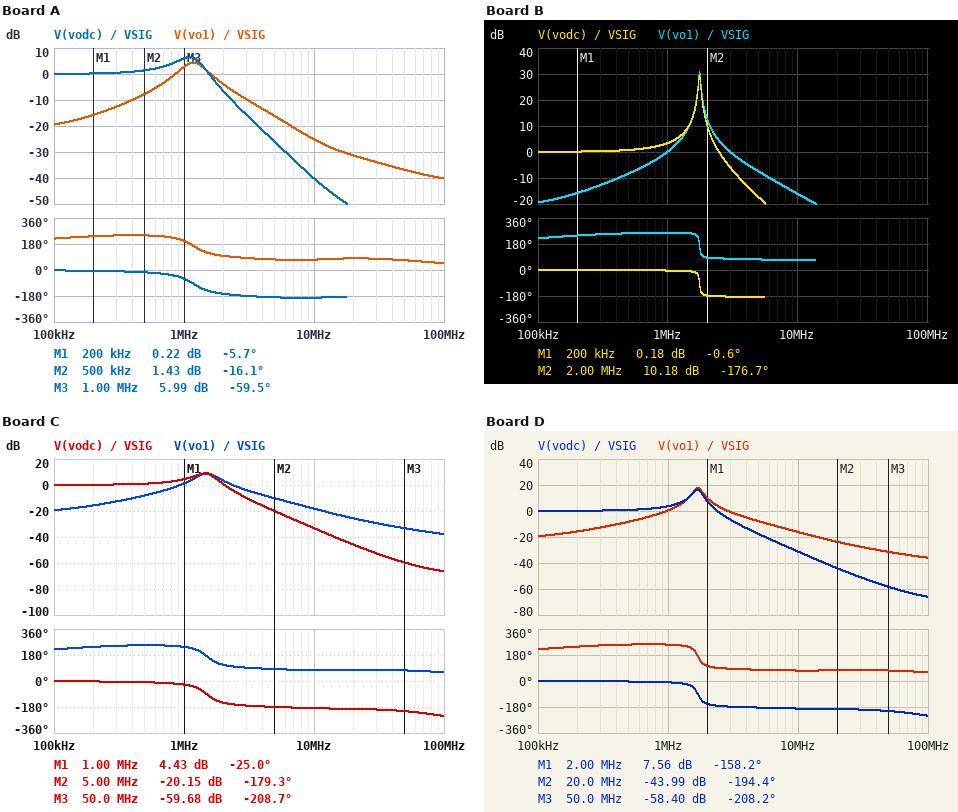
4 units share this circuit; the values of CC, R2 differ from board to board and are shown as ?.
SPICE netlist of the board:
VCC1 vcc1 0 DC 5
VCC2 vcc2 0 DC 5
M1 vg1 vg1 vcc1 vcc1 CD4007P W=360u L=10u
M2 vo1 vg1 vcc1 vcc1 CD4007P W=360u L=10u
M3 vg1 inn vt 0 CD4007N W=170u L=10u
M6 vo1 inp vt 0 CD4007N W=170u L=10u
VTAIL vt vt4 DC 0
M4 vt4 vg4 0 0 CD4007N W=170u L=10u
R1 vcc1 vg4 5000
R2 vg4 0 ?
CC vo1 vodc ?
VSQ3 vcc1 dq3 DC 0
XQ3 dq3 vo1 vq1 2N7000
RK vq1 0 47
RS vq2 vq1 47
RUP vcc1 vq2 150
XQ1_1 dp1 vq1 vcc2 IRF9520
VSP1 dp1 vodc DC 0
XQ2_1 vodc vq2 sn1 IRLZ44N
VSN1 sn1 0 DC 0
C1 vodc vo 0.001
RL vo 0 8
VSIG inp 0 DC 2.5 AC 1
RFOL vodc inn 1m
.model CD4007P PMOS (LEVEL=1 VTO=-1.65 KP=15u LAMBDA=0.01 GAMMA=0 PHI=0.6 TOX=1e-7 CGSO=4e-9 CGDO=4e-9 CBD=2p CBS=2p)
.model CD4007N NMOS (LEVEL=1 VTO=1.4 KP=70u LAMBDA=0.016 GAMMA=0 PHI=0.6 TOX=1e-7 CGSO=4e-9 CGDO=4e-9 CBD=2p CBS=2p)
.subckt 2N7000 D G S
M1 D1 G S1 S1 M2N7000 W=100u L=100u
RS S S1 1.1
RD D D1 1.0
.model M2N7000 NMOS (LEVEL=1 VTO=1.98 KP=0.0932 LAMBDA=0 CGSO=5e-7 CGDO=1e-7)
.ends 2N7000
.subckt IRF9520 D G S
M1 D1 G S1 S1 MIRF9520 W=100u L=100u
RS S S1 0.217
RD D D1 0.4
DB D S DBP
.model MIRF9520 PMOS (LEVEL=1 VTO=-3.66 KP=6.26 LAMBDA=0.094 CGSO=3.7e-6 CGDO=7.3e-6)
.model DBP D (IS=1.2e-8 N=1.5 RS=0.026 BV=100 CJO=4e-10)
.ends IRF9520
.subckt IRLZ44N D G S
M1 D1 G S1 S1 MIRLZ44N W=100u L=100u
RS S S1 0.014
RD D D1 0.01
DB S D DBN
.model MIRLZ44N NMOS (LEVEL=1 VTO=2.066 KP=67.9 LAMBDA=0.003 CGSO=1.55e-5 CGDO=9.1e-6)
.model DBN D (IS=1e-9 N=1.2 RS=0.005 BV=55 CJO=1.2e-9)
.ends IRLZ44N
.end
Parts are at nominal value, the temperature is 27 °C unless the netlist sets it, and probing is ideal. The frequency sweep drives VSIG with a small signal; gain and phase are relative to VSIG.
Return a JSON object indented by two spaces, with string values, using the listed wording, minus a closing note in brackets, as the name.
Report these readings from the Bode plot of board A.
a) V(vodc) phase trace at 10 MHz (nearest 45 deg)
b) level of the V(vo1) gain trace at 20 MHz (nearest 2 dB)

{
  "V(vodc) phase trace at 10 MHz": "-180 deg",
  "level of the V(vo1) gain trace at 20 MHz": "-32 dB"
}
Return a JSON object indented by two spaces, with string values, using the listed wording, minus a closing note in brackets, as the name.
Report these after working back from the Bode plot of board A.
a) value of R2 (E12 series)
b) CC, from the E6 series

{
  "value of R2": "3.3 kΩ",
  "CC, from the E6 series": "33 pF"
}
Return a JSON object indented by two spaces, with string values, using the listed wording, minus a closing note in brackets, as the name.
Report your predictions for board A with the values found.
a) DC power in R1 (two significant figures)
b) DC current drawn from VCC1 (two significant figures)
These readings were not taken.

{
  "DC power in R1": "1.8 mW",
  "DC current drawn from VCC1": "26 mA"
}
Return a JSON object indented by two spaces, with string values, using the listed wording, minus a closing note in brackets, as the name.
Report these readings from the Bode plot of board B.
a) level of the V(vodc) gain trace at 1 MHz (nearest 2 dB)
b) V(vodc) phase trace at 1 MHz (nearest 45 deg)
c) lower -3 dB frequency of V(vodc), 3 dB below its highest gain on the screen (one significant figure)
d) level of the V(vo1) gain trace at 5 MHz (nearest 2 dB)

{
  "level of the V(vodc) gain trace at 1 MHz": "4 dB",
  "V(vodc) phase trace at 1 MHz": "0 deg",
  "lower -3 dB frequency of V(vodc), 3 dB below its highest gain on the screen": "2 MHz",
  "level of the V(vo1) gain trace at 5 MHz": "-8 dB"
}
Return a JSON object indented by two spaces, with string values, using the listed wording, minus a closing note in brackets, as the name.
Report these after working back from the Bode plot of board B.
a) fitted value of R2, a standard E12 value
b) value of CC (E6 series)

{
  "fitted value of R2, a standard E12 value": "4.7 kΩ",
  "value of CC": "6.8 pF"
}
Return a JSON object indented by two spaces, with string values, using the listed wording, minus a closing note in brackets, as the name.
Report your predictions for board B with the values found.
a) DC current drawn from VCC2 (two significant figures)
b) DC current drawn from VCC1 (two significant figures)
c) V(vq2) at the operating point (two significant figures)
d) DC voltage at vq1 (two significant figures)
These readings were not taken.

{
  "DC current drawn from VCC2": "60 mA",
  "DC current drawn from VCC1": "27 mA",
  "V(vq2) at the operating point": "2.1 V",
  "DC voltage at vq1": "1.2 V"
}
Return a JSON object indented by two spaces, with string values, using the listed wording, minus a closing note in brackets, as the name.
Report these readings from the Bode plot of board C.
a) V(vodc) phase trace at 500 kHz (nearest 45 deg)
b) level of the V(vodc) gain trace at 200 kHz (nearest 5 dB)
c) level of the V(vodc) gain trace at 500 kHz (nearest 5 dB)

{
  "V(vodc) phase trace at 500 kHz": "0 deg",
  "level of the V(vodc) gain trace at 200 kHz": "0 dB",
  "level of the V(vodc) gain trace at 500 kHz": "0 dB"
}
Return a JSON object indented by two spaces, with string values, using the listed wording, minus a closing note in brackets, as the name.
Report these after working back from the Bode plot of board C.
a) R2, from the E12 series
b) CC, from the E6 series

{
  "R2, from the E12 series": "5.6 kΩ",
  "CC, from the E6 series": "33 pF"
}
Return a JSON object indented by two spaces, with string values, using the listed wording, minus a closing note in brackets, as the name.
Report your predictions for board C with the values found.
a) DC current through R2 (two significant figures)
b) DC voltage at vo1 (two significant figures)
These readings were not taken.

{
  "DC current through R2": "470 µA",
  "DC voltage at vo1": "3.6 V"
}
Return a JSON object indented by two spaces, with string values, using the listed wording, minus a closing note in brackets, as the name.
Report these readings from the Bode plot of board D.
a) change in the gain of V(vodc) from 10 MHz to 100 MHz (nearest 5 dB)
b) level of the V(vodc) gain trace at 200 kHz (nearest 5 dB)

{
  "change in the gain of V(vodc) from 10 MHz to 100 MHz": "-35 dB",
  "level of the V(vodc) gain trace at 200 kHz": "0 dB"
}
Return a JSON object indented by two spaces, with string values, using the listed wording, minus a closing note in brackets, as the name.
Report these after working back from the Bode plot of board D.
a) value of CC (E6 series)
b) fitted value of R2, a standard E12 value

{
  "value of CC": "15 pF",
  "fitted value of R2, a standard E12 value": "5.6 kΩ"
}
